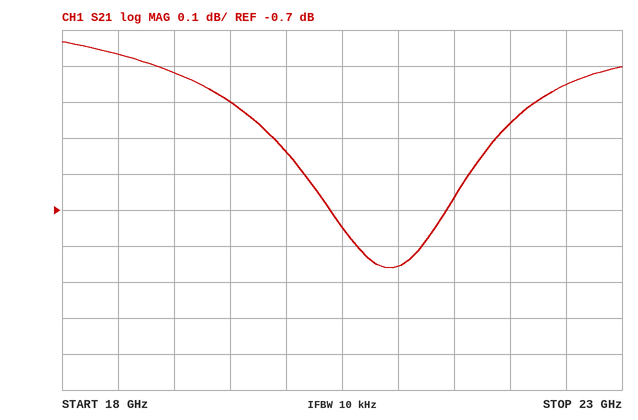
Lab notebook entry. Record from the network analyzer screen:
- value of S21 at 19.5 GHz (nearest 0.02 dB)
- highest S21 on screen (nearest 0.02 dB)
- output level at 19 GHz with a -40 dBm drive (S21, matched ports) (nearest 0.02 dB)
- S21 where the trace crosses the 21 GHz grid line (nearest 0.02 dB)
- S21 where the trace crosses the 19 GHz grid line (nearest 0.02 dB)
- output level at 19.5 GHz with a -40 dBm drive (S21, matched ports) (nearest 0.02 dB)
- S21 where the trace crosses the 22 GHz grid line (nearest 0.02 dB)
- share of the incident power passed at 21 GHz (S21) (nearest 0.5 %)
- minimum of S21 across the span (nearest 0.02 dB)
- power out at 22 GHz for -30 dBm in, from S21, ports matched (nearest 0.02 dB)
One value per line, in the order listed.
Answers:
-0.40 dB
-0.24 dB
-40.32 dBm
-0.86 dB
-0.32 dB
-40.40 dBm
-0.46 dB
82.0 %
-0.86 dB
-30.46 dBm
